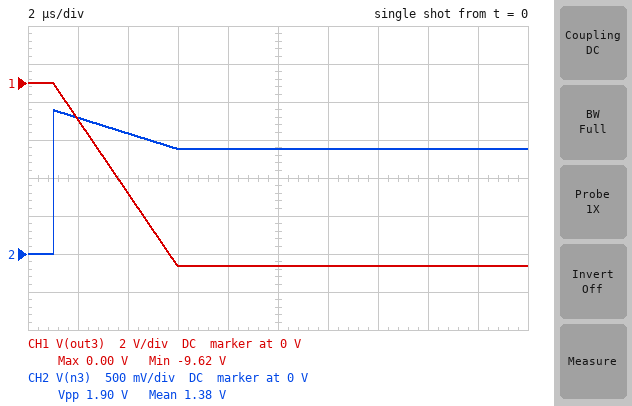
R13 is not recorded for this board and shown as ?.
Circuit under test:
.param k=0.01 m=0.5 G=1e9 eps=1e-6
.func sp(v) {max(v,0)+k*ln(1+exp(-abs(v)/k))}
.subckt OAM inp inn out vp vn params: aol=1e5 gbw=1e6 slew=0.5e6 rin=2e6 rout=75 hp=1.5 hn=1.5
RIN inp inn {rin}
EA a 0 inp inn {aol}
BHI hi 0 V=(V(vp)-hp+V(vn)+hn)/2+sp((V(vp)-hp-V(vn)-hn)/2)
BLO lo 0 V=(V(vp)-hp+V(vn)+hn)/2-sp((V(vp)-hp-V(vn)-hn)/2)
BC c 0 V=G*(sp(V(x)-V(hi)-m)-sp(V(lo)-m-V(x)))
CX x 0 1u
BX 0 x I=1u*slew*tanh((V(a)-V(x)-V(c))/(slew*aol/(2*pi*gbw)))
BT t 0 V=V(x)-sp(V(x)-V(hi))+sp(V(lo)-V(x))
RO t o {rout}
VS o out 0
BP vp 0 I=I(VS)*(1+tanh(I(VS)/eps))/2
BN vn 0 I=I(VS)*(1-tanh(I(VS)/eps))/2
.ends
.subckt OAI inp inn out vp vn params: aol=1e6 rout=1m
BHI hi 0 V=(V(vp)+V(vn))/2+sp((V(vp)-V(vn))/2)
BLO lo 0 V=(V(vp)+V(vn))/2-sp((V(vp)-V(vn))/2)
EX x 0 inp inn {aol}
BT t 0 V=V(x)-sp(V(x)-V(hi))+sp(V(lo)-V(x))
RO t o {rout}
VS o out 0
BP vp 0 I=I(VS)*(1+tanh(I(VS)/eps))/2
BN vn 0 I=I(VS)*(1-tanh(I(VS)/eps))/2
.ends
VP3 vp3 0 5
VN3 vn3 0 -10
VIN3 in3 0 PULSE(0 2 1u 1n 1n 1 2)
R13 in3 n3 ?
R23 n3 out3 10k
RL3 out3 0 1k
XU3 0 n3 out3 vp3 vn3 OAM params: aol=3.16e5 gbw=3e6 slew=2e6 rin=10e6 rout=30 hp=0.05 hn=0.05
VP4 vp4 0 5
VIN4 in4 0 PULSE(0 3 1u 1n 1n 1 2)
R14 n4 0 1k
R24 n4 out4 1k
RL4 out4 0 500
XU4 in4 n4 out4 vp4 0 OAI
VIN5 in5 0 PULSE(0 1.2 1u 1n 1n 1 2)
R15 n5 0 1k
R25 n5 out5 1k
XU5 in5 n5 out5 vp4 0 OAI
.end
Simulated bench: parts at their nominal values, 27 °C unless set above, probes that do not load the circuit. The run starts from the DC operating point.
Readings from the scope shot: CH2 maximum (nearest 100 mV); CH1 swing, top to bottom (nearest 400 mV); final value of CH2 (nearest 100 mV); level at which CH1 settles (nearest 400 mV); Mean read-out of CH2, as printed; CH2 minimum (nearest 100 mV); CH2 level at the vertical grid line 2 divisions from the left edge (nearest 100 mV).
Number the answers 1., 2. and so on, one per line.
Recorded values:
1. 1.9 V
2. 9.6 V
3. 1.4 V
4. -9.6 V
5. 1.38 V
6. 0 V
7. 1.6 V
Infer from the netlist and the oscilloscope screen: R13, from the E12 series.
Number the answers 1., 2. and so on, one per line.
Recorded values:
1. 560 Ω
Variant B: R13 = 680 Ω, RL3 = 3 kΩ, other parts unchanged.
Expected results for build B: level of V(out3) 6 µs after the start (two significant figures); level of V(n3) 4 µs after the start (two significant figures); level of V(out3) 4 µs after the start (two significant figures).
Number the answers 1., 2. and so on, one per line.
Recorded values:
1. -9.8 V
2. 1.5 V
3. -5.9 V
